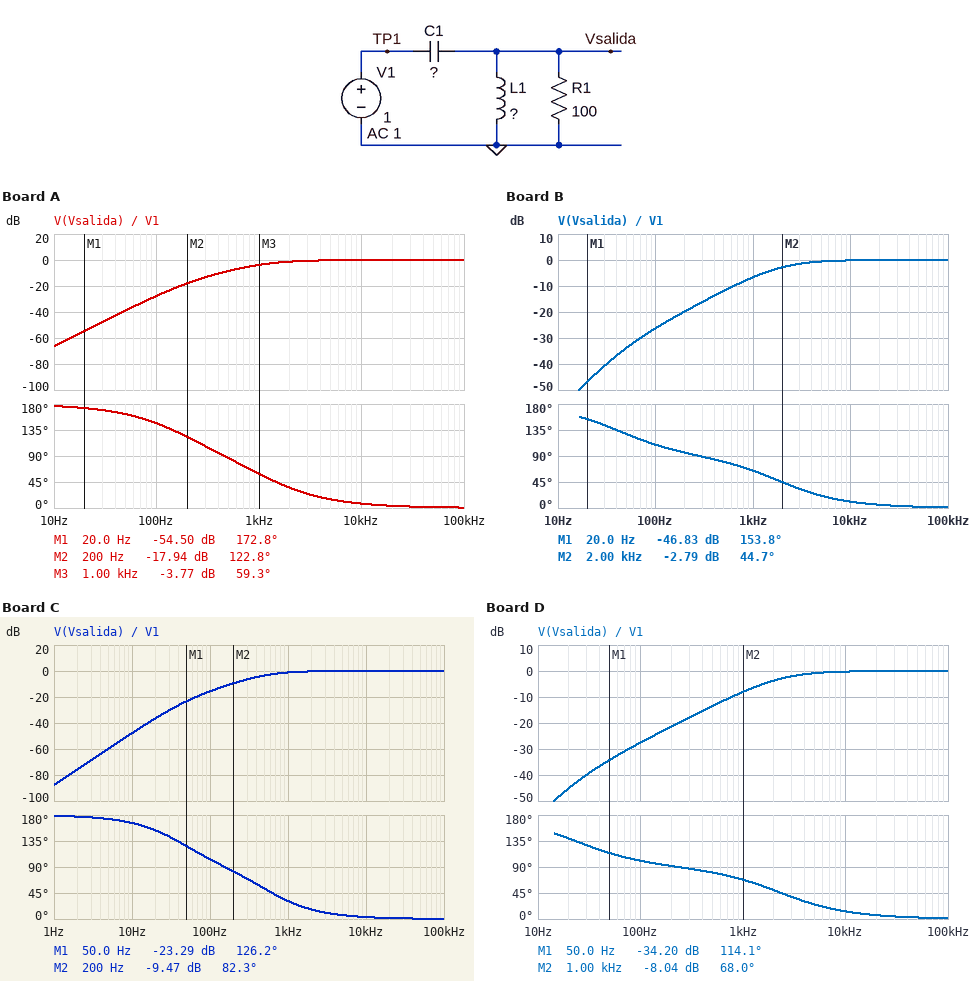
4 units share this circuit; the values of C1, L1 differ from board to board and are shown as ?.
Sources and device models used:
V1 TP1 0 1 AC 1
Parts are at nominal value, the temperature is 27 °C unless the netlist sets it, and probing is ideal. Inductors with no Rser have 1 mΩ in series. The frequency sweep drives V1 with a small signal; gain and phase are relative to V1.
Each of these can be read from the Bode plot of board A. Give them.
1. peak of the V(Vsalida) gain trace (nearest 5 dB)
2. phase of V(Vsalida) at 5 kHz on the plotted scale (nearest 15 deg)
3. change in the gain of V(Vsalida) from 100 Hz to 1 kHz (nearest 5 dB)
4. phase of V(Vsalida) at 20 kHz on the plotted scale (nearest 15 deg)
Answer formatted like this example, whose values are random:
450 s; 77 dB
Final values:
0 dB; 15 deg; 25 dB; 0 deg
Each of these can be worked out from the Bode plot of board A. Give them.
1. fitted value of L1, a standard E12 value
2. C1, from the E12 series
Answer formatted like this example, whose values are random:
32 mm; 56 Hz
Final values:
100 mH; 1.2 µF
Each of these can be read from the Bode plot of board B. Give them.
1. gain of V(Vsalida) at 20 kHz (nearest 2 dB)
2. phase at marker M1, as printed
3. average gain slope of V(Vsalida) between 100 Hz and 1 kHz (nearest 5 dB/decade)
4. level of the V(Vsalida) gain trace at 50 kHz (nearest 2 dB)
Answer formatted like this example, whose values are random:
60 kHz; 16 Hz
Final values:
0 dB; 153.8 deg; 20 dB/decade; 0 dB
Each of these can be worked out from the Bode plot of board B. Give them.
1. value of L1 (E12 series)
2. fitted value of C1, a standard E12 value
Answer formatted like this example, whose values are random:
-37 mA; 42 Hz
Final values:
390 mH; 820 nF
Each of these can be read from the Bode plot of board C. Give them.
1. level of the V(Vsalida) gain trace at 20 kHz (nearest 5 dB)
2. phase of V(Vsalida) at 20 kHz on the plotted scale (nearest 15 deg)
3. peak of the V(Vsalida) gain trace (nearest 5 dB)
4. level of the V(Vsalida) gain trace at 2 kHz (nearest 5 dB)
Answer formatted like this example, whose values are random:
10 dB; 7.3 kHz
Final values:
0 dB; 0 deg; 0 dB; 0 dB
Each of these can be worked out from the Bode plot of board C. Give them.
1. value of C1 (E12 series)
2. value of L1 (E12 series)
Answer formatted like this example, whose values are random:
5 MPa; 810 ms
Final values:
2.7 µF; 390 mH
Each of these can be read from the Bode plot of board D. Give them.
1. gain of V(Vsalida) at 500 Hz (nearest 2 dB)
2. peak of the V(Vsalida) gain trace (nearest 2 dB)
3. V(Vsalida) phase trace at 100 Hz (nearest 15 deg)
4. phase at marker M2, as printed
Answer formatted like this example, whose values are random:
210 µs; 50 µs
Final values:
-14 dB; 0 dB; 105 deg; 68.0 deg
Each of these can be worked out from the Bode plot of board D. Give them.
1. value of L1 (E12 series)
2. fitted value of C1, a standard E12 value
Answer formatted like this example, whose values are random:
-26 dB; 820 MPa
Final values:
680 mH; 680 nF
